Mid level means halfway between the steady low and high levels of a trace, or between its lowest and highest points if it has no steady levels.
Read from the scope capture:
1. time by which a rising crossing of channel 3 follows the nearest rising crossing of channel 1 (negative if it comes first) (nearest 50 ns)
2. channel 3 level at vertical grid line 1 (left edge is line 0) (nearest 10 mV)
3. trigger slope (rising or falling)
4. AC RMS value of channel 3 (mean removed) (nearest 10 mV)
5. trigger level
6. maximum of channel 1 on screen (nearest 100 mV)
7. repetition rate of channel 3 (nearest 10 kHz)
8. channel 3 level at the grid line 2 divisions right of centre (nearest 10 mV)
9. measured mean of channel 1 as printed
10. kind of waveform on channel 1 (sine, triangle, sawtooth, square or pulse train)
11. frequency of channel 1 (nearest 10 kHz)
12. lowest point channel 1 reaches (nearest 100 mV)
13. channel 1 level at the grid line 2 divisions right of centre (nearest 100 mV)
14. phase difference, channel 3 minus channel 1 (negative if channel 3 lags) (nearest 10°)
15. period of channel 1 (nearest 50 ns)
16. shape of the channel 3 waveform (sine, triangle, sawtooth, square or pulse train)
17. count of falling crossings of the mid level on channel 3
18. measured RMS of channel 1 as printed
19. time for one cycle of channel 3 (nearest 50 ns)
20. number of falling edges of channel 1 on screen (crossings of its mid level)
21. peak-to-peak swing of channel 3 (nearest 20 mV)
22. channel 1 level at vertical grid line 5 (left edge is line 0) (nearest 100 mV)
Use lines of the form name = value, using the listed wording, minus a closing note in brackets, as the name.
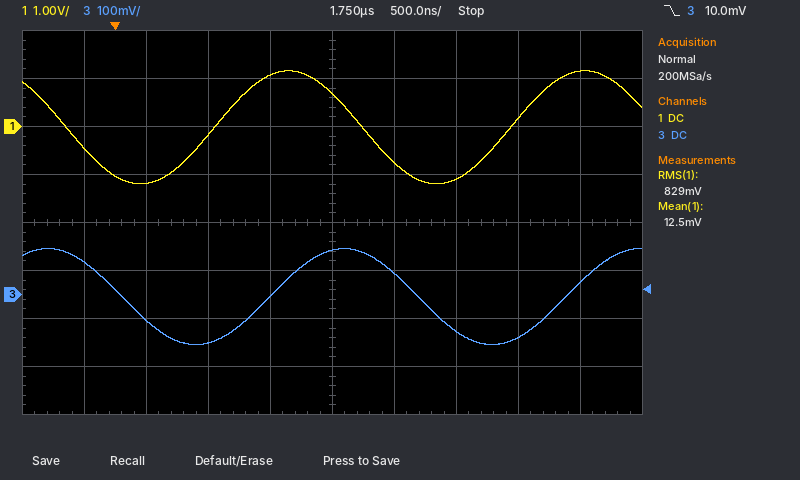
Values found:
time by which a rising crossing of channel 3 follows the nearest rising crossing of channel 1 (negative if it comes first) = +450 ns
channel 3 level at vertical grid line 1 (left edge is line 0) = 70 mV
trigger slope = falling
AC RMS value of channel 3 (mean removed) = 70 mV
trigger level = 10.0 mV
maximum of channel 1 on screen = 1.2 V
repetition rate of channel 3 = 420 kHz
channel 3 level at the grid line 2 divisions right of centre = -80 mV
measured mean of channel 1 as printed = 12.5 mV
kind of waveform on channel 1 = sine
frequency of channel 1 = 420 kHz
lowest point channel 1 reaches = -1.2 V
channel 1 level at the grid line 2 divisions right of centre = -1.1 V
phase difference, channel 3 minus channel 1 (negative if channel 3 lags) = -70°
period of channel 1 = 2.40 µs
shape of the channel 3 waveform = sine
count of falling crossings of the mid level on channel 3 = 2
measured RMS of channel 1 as printed = 829 mV
time for one cycle of channel 3 = 2.40 µs
number of falling edges of channel 1 on screen = 2
peak-to-peak swing of channel 3 = 200 mV
channel 1 level at vertical grid line 5 (left edge is line 0) = 700 mV
